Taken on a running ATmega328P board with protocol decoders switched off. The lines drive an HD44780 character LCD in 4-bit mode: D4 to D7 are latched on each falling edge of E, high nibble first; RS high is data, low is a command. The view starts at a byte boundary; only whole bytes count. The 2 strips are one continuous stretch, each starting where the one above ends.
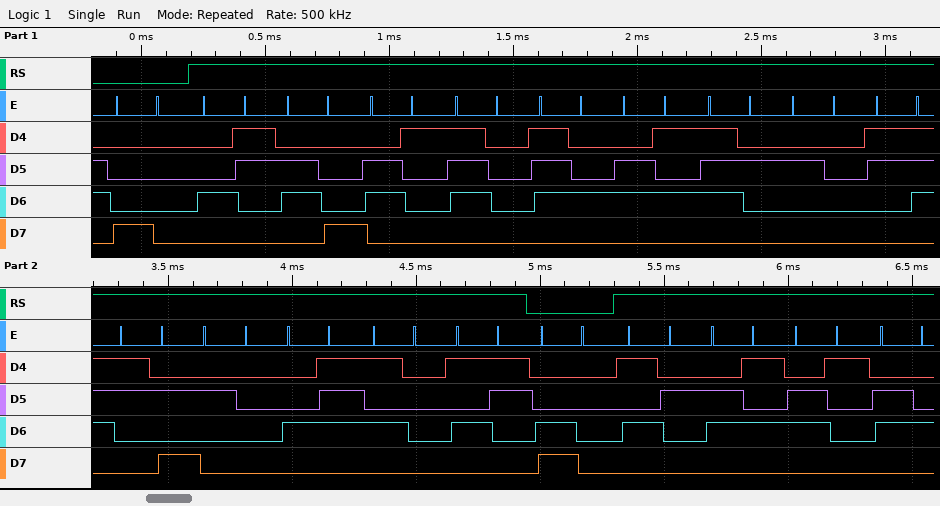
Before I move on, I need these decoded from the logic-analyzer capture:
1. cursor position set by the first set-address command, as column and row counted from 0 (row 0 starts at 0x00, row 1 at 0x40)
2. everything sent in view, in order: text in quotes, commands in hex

column 0, row 0
0x80 "Chapter 7: GPS" 0xC0 "Read"
